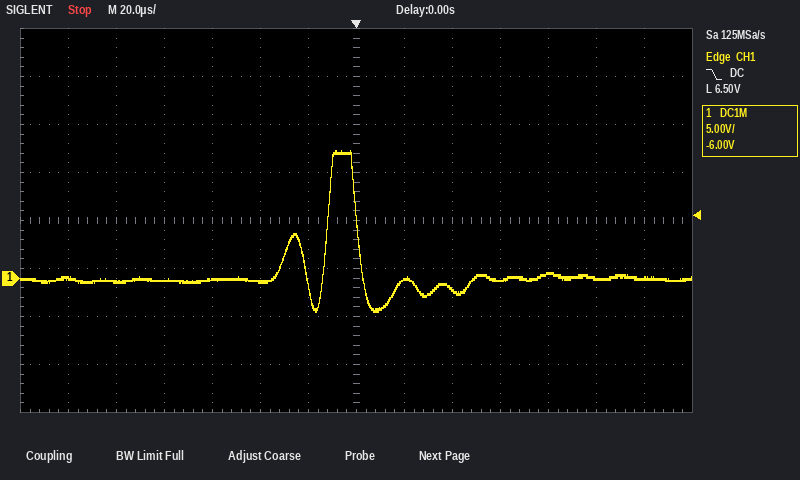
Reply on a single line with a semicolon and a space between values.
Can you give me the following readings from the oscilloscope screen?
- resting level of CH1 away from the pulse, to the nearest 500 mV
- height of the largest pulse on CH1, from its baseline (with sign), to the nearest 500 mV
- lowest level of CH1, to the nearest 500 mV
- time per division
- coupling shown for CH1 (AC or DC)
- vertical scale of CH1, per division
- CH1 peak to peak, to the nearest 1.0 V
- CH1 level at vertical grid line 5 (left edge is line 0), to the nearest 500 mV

0.0 V; +13.5 V; -3.5 V; 20 µs; DC; 5 V; 17.0 V; -500 mV
